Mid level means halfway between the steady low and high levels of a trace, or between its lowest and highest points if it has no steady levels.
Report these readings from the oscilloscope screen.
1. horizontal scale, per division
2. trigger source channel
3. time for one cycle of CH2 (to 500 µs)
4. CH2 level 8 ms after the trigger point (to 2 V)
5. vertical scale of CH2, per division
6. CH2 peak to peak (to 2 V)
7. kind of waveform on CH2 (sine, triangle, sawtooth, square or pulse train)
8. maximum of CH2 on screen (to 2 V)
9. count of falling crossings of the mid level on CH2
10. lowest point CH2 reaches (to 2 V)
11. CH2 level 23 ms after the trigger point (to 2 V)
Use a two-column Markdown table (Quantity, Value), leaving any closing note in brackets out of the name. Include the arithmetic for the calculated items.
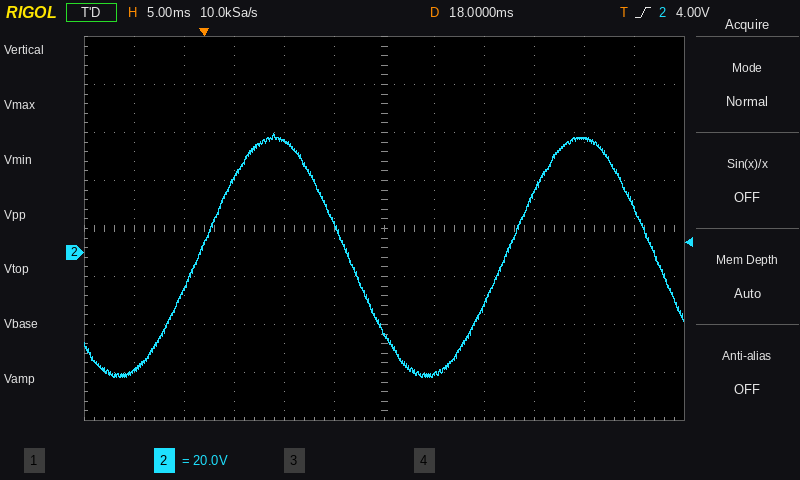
| Quantity | Value |
|---|---|
| horizontal scale, per division | 5 ms |
| trigger source channel | CH2 |
| time for one cycle of CH2 | 30.5 ms |
| CH2 level 8 ms after the trigger point | 46 V |
| vertical scale of CH2, per division | 20 V |
| CH2 peak to peak | 50 V − (-52 V) = 102 V |
| kind of waveform on CH2 | sine |
| maximum of CH2 on screen | 50 V |
| count of falling crossings of the mid level on CH2 | 2 |
| lowest point CH2 reaches | -52 V |
| CH2 level 23 ms after the trigger point | -50 V |
